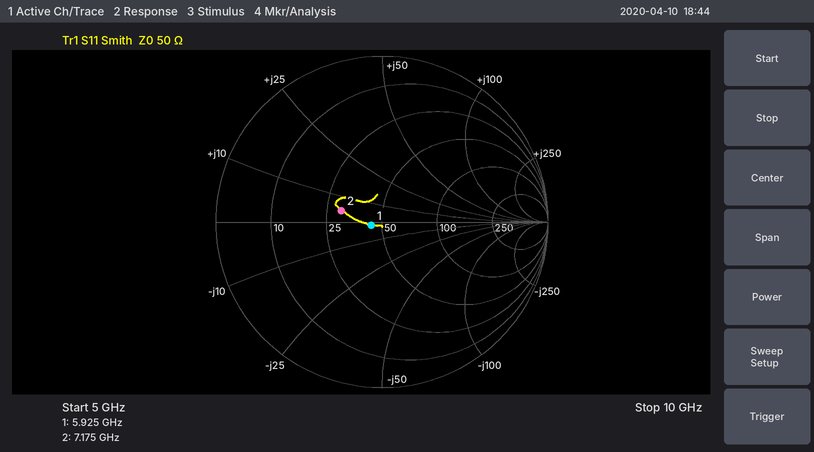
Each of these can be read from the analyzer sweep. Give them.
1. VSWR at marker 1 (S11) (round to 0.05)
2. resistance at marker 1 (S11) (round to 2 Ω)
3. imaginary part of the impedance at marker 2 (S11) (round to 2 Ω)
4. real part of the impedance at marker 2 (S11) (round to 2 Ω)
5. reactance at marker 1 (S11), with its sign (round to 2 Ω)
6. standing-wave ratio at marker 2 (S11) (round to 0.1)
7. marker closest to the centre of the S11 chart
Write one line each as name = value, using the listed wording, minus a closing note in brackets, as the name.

VSWR at marker 1 (S11) = 1.15
resistance at marker 1 (S11) = 44 Ω
imaginary part of the impedance at marker 2 (S11) = +4 Ω
real part of the impedance at marker 2 (S11) = 30 Ω
reactance at marker 1 (S11), with its sign = -2 Ω
standing-wave ratio at marker 2 (S11) = 1.7
marker closest to the centre of the S11 chart = marker 1
